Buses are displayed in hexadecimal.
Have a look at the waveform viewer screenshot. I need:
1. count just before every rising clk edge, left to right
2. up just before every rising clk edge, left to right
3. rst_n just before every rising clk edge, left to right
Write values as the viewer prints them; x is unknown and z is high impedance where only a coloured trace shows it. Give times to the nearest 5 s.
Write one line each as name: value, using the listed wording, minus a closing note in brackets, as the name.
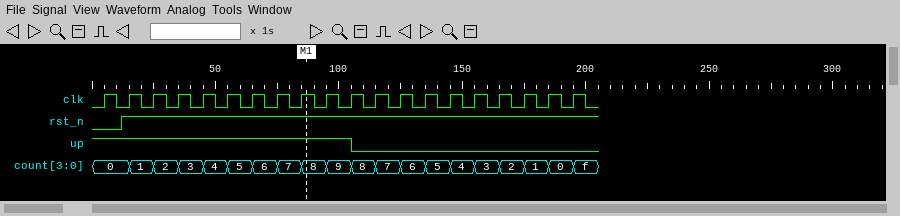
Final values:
count just before every rising clk edge, left to right: 0, 0, 1, 2, 3, 4, 5, 6, 7, 8, 9, 8, 7, 6, 5, 4, 3, 2, 1, 0
up just before every rising clk edge, left to right: 1 1 1 1 1 1 1 1 1 1 1 0 0 0 0 0 0 0 0 0
rst_n just before every rising clk edge, left to right: 0 1 1 1 1 1 1 1 1 1 1 1 1 1 1 1 1 1 1 1
